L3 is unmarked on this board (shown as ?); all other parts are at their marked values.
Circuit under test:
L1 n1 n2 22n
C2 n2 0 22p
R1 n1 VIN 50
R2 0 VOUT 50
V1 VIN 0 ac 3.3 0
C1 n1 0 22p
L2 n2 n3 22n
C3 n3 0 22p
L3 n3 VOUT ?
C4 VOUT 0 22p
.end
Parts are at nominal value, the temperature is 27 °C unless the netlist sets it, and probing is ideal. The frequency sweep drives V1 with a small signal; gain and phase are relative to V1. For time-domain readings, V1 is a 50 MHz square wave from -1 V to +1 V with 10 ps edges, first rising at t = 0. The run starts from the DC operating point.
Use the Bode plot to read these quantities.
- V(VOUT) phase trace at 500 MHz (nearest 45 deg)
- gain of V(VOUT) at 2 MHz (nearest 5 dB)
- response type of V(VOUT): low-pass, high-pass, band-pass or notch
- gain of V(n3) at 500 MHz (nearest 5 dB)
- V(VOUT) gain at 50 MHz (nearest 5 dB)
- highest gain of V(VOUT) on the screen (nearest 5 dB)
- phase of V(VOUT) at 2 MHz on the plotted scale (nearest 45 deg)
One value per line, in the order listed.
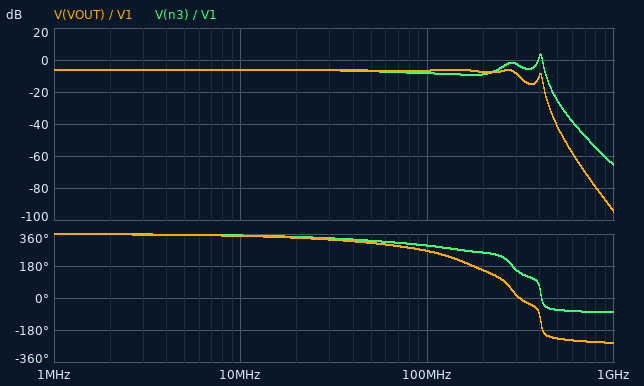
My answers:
-225 deg
-5 dB
low-pass
-25 dB
-5 dB
-5 dB
360 deg
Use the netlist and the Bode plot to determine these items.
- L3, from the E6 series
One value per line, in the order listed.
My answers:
33 nH
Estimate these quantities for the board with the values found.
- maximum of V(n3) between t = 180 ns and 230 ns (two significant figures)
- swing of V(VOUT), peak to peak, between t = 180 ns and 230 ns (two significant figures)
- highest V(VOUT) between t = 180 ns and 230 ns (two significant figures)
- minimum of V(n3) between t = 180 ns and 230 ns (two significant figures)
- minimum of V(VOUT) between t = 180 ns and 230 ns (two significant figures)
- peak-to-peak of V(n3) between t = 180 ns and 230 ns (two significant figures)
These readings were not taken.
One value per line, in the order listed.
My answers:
580 mV
1.2 V
580 mV
-580 mV
-580 mV
1.2 V
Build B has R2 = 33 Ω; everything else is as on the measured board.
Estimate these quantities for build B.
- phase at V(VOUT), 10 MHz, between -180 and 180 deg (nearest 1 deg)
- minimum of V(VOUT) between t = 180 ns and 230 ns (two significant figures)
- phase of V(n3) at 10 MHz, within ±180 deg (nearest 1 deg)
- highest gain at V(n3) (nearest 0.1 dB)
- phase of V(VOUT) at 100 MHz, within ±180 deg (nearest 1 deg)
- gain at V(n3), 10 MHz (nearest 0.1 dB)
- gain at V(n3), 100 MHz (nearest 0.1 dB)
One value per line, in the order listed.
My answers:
-10 deg
-490 mV
-6 deg
3.2 dB
-97 deg
-8.0 dB
-8.4 dB
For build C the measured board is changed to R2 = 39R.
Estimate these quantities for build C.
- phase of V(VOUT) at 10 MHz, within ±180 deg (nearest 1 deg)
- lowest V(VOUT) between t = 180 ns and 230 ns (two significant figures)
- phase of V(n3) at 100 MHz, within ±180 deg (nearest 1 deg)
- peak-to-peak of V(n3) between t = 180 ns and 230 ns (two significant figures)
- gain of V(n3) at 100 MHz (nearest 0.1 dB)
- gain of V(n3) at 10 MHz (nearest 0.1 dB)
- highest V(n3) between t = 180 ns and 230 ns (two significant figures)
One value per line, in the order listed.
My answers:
-10 deg
-530 mV
-60 deg
1.1 V
-8.4 dB
-7.2 dB
550 mV
